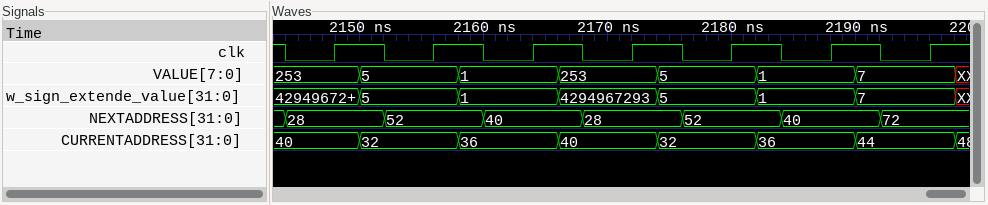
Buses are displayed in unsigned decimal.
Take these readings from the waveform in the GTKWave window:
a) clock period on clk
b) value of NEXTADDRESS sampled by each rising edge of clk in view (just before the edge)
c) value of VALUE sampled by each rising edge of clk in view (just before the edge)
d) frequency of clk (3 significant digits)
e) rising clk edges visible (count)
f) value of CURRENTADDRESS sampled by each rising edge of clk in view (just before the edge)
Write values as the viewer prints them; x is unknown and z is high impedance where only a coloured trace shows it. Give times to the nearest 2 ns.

8 ns
28, 52, 40, 28, 52, 40, 72
253, 5, 1, 253, 5, 1, 7
125 MHz
7
40, 32, 36, 40, 32, 36, 44
